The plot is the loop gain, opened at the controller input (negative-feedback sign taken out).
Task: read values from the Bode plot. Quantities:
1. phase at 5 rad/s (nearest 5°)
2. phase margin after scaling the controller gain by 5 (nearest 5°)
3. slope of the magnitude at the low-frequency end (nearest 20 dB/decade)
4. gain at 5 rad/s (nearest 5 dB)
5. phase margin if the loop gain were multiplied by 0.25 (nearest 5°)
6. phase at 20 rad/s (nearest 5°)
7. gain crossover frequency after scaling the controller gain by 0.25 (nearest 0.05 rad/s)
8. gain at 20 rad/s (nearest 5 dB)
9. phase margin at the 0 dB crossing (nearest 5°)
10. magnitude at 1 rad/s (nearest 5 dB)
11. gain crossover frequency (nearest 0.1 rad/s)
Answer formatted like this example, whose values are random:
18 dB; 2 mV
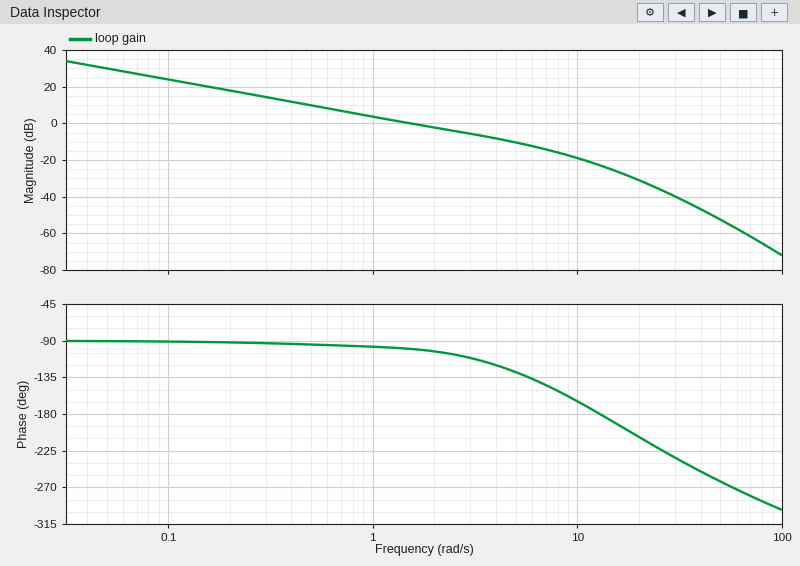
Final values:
-130°; 35°; -20 dB/decade; -10 dB; 85°; -210°; 0.40 rad/s; -30 dB; 80°; 5 dB; 1.5 rad/s
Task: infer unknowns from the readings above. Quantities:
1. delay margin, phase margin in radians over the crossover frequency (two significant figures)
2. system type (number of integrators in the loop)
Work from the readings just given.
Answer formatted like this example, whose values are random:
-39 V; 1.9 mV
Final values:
0.93 s; 1
